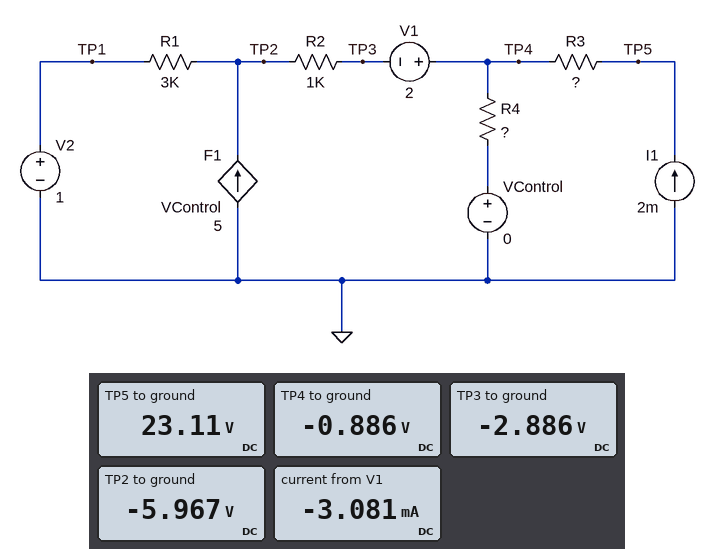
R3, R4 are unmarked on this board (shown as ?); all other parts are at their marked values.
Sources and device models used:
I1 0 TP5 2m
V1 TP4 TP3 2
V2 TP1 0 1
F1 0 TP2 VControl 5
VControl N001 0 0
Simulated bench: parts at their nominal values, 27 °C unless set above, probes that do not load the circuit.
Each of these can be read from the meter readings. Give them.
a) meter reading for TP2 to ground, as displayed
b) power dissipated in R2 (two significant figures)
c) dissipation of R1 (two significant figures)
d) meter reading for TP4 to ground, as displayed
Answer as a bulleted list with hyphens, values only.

- -5.967 V
- 9.5 mW
- 16 mW
- -0.886 V
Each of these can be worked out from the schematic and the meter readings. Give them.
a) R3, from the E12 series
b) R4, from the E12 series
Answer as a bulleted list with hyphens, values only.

- 12 kΩ
- 820 Ω
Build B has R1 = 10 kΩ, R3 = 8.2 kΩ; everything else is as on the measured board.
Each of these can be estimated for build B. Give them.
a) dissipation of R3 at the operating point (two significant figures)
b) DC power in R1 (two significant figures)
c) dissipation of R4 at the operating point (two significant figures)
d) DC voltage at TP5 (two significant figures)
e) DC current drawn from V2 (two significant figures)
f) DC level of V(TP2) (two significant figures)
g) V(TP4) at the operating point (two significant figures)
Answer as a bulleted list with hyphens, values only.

- 33 mW
- 3.8 mW
- 350 µW
- 16 V
- 620 µA
- -5.2 V
- -540 mV
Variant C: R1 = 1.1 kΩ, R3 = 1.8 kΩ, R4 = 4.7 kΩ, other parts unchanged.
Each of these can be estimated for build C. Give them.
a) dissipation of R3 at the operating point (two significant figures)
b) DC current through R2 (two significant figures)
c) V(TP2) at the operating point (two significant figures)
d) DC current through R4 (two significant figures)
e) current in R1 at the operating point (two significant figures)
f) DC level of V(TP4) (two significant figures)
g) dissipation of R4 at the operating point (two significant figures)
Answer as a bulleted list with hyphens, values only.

- 7.2 mW
- 3.5 mA
- 28 V
- 5.5 mA
- 24 mA
- 26 V
- 140 mW
